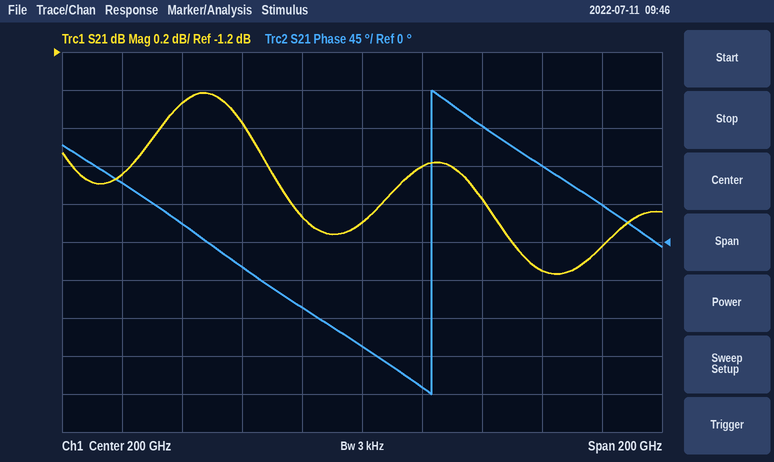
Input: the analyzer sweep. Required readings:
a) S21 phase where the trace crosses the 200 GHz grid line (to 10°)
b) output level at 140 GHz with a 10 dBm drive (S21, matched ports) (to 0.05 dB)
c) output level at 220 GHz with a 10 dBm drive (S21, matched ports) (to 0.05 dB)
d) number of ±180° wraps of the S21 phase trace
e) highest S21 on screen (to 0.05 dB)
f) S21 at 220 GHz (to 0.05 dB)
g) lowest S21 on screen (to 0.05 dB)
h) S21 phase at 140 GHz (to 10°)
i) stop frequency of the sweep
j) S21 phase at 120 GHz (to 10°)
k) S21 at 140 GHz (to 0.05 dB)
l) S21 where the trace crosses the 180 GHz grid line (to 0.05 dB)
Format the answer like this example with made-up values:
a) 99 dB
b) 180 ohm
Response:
a) -120°
b) 8.55 dBm
c) 8.20 dBm
d) 1
e) -1.40 dB
f) -1.80 dB
g) -2.35 dB
h) 20°
i) 300 GHz
j) 70°
k) -1.45 dB
l) -2.05 dB
